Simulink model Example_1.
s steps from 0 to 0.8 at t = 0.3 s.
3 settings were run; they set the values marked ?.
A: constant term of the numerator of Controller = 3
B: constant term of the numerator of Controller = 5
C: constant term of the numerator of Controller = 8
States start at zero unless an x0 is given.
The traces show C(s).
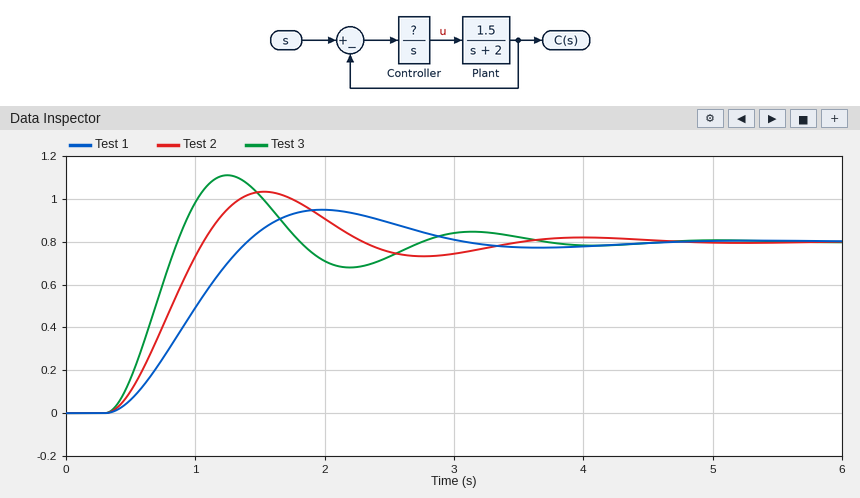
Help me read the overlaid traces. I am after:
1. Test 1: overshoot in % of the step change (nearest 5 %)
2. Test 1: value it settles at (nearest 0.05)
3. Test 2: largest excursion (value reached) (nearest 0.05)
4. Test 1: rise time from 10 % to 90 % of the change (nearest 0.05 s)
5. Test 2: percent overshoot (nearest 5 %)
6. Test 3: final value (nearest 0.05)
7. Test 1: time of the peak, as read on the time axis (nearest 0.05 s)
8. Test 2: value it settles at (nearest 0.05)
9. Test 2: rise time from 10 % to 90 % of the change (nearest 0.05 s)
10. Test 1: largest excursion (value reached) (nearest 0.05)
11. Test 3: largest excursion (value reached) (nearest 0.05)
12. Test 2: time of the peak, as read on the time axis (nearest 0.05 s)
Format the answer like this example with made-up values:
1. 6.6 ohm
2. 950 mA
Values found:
1. 20 %
2. 0.80
3. 1.05
4. 0.75 s
5. 30 %
6. 0.80
7. 2.00 s
8. 0.80
9. 0.50 s
10. 0.95
11. 1.10
12. 1.55 s
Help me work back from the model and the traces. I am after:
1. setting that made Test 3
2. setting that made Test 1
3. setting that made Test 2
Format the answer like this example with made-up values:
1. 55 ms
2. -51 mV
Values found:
1. C
2. A
3. B
